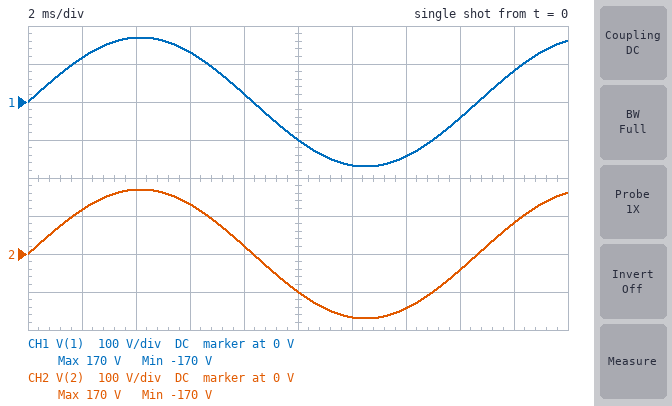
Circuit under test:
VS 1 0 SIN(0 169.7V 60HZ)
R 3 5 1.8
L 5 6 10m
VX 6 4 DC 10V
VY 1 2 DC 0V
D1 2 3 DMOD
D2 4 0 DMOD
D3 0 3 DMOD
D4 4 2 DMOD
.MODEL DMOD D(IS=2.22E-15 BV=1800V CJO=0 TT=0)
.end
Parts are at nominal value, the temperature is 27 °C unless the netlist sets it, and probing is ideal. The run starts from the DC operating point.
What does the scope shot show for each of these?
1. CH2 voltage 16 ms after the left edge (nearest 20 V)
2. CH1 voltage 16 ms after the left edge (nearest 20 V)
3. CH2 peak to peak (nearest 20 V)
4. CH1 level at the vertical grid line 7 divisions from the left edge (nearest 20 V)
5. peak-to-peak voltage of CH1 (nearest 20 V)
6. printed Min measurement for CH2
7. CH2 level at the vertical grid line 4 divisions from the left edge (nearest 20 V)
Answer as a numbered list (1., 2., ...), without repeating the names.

1. -40 V
2. -40 V
3. 340 V
4. -140 V
5. 340 V
6. -170 V
7. 20 V
